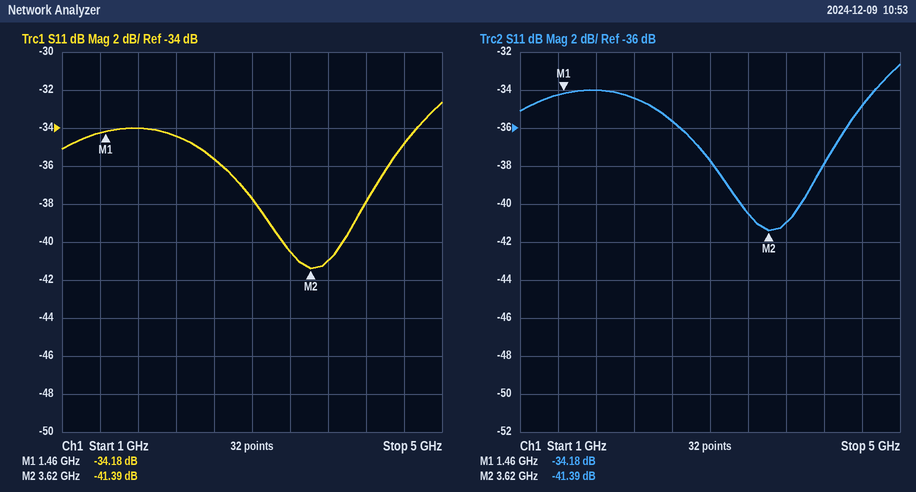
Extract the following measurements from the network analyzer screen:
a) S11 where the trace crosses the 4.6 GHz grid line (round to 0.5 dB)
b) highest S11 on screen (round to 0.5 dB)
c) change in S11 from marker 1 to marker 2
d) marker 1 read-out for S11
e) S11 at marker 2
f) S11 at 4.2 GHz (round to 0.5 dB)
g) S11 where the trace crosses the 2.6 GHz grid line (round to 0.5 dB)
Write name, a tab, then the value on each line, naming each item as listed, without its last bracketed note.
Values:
S11 where the trace crosses the 4.6 GHz grid line	-35.0 dB
highest S11 on screen	-32.5 dB
change in S11 from marker 1 to marker 2	-7.21 dB
marker 1 read-out for S11	-34.18 dB
S11 at marker 2	-41.39 dB
S11 at 4.2 GHz	-38.0 dB
S11 where the trace crosses the 2.6 GHz grid line	-35.5 dB
